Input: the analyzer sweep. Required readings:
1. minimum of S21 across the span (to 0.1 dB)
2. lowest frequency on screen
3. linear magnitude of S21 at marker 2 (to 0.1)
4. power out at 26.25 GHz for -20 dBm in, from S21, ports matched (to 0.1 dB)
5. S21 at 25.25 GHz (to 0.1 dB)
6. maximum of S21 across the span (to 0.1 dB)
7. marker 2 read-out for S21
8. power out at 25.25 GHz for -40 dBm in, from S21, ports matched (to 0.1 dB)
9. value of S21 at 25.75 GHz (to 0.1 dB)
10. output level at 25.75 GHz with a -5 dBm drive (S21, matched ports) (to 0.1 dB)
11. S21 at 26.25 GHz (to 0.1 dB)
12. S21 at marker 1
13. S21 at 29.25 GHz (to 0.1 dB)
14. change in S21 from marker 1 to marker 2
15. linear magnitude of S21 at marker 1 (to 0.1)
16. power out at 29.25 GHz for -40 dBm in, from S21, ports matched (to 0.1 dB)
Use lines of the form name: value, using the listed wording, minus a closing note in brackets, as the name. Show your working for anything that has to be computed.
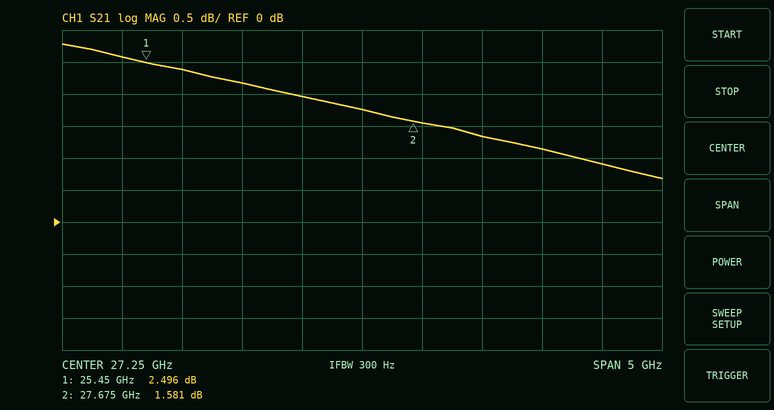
minimum of S21 across the span: 0.7 dB
lowest frequency on screen: 24.75 GHz
linear magnitude of S21 at marker 2: 10^(1.581/20) ≈ 1.2
power out at 26.25 GHz for -20 dBm in, from S21, ports matched: -20 dBm + (2.2 dB) = -17.8 dBm
S21 at 25.25 GHz: 2.6 dB
maximum of S21 across the span: 2.8 dB
marker 2 read-out for S21: 1.581 dB
power out at 25.25 GHz for -40 dBm in, from S21, ports matched: -40 dBm + (2.6 dB) = -37.4 dBm
value of S21 at 25.75 GHz: 2.4 dB
output level at 25.75 GHz with a -5 dBm drive (S21, matched ports): -5 dBm + (2.4 dB) = -2.6 dBm
S21 at 26.25 GHz: 2.2 dB
S21 at marker 1: 2.496 dB
S21 at 29.25 GHz: 0.9 dB
change in S21 from marker 1 to marker 2: 1.581 − (2.496) = -0.915 dB
linear magnitude of S21 at marker 1: 10^(2.496/20) ≈ 1.3
power out at 29.25 GHz for -40 dBm in, from S21, ports matched: -40 dBm + (0.9 dB) = -39.1 dBm
